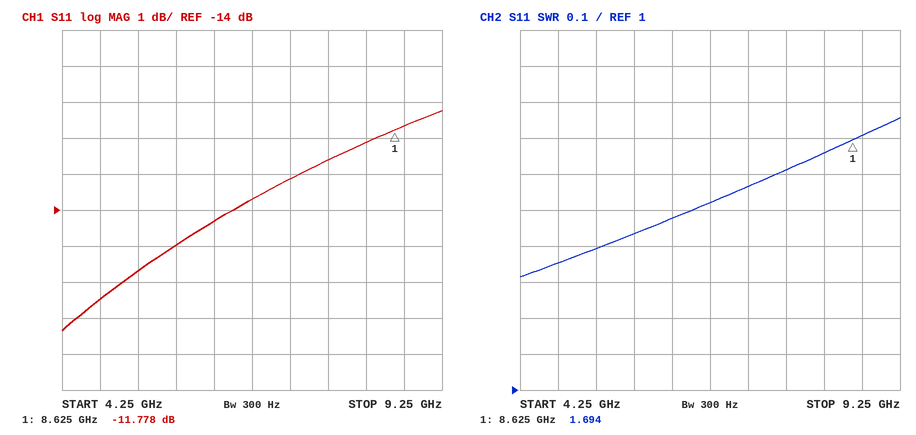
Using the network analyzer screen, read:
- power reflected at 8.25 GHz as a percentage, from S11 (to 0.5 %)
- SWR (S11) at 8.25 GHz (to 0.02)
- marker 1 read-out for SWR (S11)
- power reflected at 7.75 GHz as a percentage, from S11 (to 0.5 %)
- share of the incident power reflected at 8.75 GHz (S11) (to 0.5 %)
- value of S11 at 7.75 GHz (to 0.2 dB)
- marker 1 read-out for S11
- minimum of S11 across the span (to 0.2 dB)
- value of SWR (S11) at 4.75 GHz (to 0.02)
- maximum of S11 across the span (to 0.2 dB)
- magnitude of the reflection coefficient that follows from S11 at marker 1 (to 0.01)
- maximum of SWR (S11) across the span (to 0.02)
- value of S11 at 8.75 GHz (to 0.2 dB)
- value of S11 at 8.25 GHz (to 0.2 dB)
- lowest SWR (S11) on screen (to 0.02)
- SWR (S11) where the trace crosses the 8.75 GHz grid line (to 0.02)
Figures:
6.0 %
1.66
1.694
5.5 %
7.0 %
-12.6 dB
-11.778 dB
-17.4 dB
1.36
-11.2 dB
0.26
1.76
-11.6 dB
-12.2 dB
1.32
1.70
